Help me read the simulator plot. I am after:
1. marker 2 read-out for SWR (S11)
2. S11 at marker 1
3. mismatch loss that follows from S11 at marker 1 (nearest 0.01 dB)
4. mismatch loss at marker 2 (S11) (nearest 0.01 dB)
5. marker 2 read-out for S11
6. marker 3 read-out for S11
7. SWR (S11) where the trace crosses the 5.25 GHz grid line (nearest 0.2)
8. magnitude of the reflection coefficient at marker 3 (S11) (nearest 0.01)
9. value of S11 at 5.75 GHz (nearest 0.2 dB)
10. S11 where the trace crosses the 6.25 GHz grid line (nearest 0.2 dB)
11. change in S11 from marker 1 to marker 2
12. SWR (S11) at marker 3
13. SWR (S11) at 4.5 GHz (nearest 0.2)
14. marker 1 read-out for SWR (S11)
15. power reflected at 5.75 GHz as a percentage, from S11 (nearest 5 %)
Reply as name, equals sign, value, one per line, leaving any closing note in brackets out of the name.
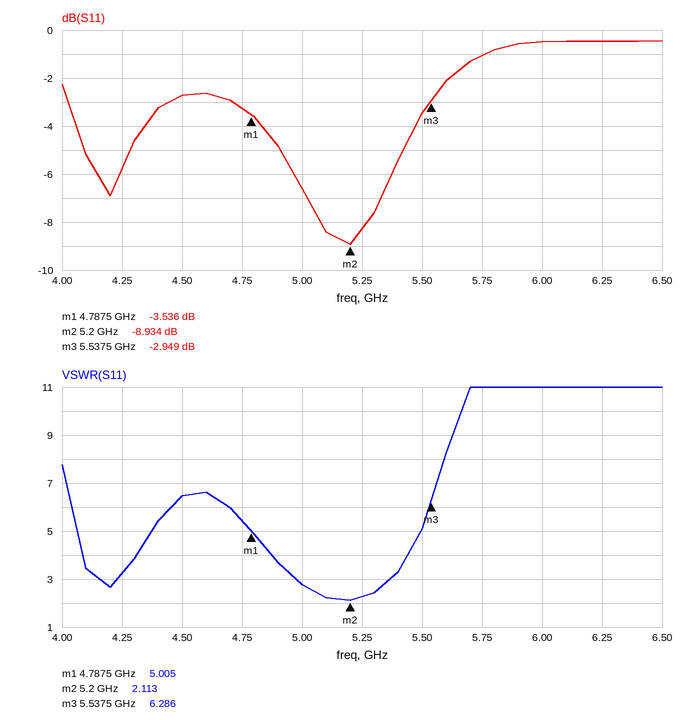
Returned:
marker 2 read-out for SWR = 2.113
S11 at marker 1 = -3.536 dB
mismatch loss that follows from S11 at marker 1 = 2.54 dB
mismatch loss at marker 2 (S11) = 0.59 dB
marker 2 read-out for S11 = -8.934 dB
marker 3 read-out for S11 = -2.949 dB
SWR (S11) where the trace crosses the 5.25 GHz grid line = 2.2
magnitude of the reflection coefficient at marker 3 (S11) = 0.71
value of S11 at 5.75 GHz = -1.0 dB
S11 where the trace crosses the 6.25 GHz grid line = -0.4 dB
change in S11 from marker 1 to marker 2 = -5.398 dB
SWR (S11) at marker 3 = 6.286
SWR (S11) at 4.5 GHz = 6.4
marker 1 read-out for SWR = 5.005
power reflected at 5.75 GHz as a percentage, from S11 = 80 %
